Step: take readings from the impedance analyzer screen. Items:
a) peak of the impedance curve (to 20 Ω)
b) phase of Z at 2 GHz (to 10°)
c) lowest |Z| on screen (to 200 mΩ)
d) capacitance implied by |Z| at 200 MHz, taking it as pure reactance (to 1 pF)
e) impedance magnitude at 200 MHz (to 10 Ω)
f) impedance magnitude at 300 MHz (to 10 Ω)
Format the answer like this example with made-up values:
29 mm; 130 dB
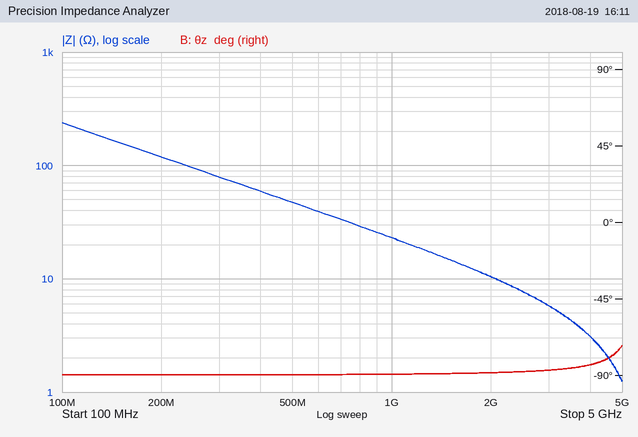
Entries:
240 Ω; -90°; 1.2 Ω; 7 pF; 120 Ω; 80 Ω
